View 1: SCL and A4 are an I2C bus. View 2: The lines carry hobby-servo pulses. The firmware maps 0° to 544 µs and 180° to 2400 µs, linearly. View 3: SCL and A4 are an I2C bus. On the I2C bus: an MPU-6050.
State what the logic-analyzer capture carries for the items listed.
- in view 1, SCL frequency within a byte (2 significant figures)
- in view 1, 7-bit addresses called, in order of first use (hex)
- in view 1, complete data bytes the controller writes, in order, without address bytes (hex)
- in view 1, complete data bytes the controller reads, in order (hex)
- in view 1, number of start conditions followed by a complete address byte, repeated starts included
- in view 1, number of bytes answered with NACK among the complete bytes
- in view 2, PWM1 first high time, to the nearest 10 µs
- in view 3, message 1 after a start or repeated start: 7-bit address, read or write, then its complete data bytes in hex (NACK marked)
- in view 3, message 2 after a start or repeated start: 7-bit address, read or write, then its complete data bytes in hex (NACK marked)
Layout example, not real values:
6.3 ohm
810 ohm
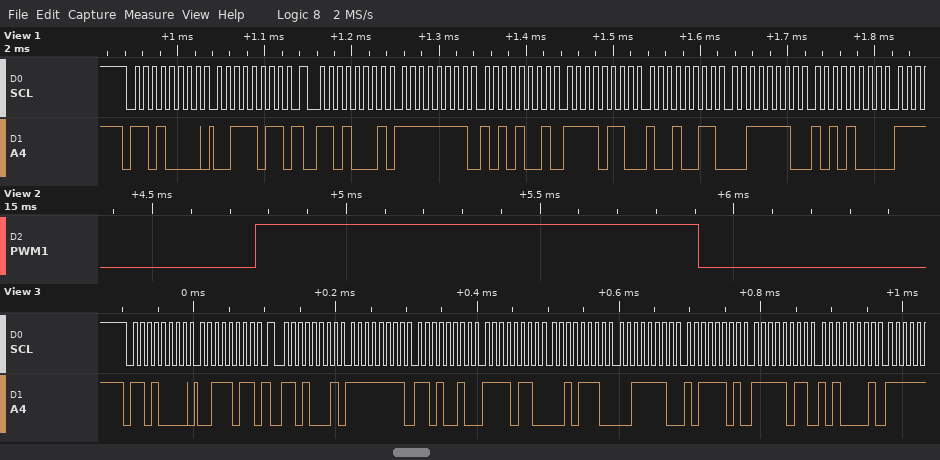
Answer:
100 kHz
0x68
3B
FF A9 F6 93 3E A8
2
0
1140 µs
0x68 write: 3B
0x68 read: FF D2 F6 2E 3E BD FB A1
